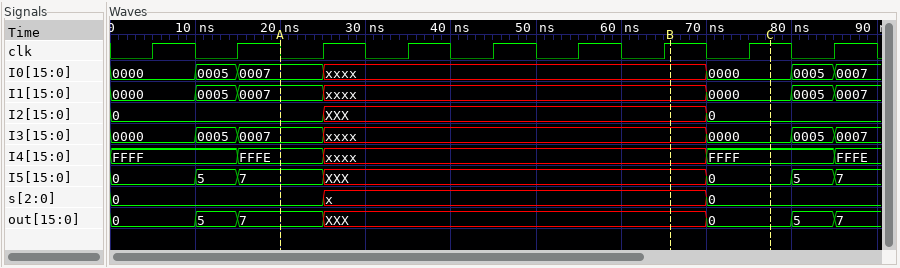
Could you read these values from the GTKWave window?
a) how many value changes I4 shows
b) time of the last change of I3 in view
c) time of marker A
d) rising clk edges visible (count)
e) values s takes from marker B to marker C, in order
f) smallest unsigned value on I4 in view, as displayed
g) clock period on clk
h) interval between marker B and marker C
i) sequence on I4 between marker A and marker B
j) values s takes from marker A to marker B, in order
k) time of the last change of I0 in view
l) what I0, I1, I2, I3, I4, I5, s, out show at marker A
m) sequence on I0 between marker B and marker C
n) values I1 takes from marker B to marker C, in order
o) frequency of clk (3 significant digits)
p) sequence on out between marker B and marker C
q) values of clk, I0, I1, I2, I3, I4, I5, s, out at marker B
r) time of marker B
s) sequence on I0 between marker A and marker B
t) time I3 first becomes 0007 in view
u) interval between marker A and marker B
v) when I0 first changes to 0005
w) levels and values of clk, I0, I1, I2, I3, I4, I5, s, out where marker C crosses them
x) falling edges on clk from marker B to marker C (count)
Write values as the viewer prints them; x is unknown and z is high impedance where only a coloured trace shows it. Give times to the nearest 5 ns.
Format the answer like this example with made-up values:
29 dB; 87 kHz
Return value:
4; 85 ns; 20 ns; 9; x, 0; FFFE; 10 ns; 10 ns; FFFE, xxxx; 0, x; 85 ns; I0=0007, I1=0007, I2=0, I3=0007, I4=FFFE, I5=7, s=0, out=7; xxxx, 0000; xxxx, 0000; 100 MHz; XXX, 0; clk=1, I0=xxxx, I1=xxxx, I2=XXX, I3=xxxx, I4=xxxx, I5=XXX, s=x, out=XXX; 65 ns; 0007, xxxx; 15 ns; 45 ns; 10 ns; clk=1, I0=0000, I1=0000, I2=0, I3=0000, I4=FFFF, I5=0, s=0, out=0; 1
